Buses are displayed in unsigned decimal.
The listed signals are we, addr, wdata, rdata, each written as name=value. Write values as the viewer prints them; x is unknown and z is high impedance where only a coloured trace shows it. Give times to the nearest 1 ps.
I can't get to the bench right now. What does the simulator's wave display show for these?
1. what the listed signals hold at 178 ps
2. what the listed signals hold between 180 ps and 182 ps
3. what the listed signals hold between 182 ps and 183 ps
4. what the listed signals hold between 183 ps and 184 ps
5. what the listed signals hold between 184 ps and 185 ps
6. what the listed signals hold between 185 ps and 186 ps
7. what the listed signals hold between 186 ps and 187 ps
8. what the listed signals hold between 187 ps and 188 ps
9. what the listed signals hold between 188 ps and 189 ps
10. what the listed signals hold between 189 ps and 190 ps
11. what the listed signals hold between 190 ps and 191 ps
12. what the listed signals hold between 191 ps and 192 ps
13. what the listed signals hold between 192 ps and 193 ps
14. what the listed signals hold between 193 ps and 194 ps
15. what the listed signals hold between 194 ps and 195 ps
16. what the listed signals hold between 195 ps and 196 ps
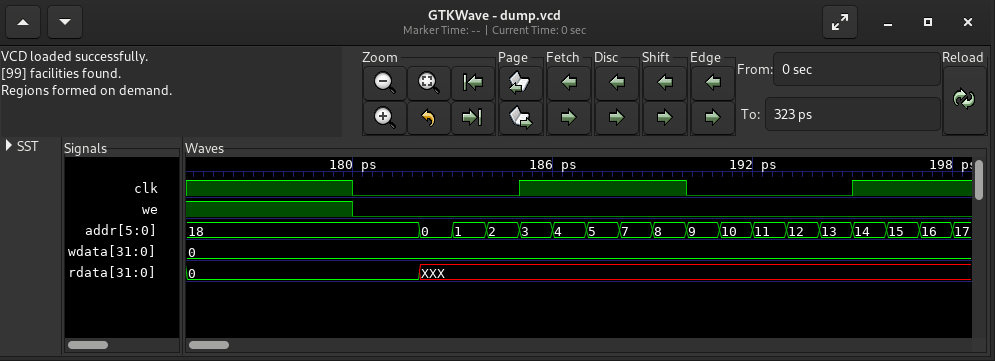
we=1, addr=18, wdata=0, rdata=0
we=0, addr=18, wdata=0, rdata=0
we=0, addr=0, wdata=0, rdata=XXX
we=0, addr=1, wdata=0, rdata=XXX
we=0, addr=2, wdata=0, rdata=XXX
we=0, addr=3, wdata=0, rdata=XXX
we=0, addr=4, wdata=0, rdata=XXX
we=0, addr=5, wdata=0, rdata=XXX
we=0, addr=7, wdata=0, rdata=XXX
we=0, addr=8, wdata=0, rdata=XXX
we=0, addr=9, wdata=0, rdata=XXX
we=0, addr=10, wdata=0, rdata=XXX
we=0, addr=11, wdata=0, rdata=XXX
we=0, addr=12, wdata=0, rdata=XXX
we=0, addr=13, wdata=0, rdata=XXX
we=0, addr=14, wdata=0, rdata=XXX
